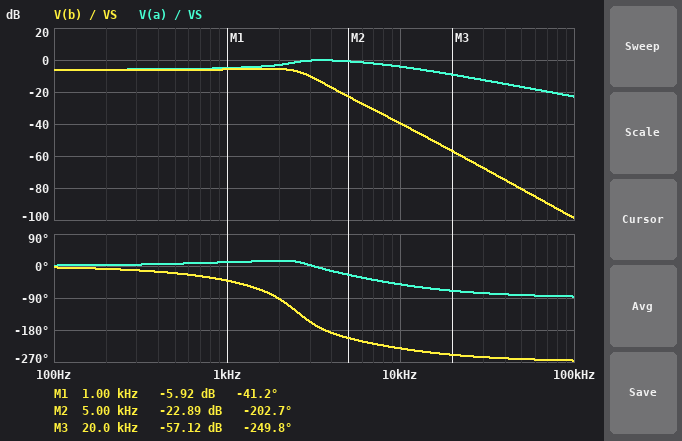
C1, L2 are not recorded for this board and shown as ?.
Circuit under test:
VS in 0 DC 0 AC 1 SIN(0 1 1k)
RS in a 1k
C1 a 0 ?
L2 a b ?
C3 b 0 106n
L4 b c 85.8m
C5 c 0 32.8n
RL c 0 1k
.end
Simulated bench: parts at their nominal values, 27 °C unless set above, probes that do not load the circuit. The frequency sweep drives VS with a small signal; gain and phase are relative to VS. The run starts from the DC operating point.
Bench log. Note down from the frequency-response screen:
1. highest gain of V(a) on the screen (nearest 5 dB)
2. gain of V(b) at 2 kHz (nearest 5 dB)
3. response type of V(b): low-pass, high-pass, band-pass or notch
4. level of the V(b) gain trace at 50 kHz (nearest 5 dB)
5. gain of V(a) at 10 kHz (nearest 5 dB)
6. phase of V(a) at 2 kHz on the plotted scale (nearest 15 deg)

0 dB
-5 dB
low-pass
-80 dB
-5 dB
15 deg
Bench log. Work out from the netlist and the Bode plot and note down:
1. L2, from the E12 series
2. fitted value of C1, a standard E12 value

150 mH
22 nF
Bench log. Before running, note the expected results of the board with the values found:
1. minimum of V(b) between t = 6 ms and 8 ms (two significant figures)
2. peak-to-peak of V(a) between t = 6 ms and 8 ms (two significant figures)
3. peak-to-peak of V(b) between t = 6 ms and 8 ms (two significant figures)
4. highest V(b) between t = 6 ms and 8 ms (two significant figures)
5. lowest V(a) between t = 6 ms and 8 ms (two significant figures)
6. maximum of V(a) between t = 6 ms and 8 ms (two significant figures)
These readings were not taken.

-510 mV
1.1 V
1.0 V
510 mV
-560 mV
560 mV
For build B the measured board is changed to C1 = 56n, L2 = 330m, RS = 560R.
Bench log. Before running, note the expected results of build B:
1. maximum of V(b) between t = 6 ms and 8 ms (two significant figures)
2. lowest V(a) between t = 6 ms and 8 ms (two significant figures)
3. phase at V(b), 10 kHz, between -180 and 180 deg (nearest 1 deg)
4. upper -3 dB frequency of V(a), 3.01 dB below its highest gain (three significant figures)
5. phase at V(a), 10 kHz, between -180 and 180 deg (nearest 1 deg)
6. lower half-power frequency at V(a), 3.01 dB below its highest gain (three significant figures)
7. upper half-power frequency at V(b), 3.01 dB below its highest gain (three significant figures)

450 mV
-880 mV
117 deg
5.88 kHz
-63 deg
223 Hz
995 Hz
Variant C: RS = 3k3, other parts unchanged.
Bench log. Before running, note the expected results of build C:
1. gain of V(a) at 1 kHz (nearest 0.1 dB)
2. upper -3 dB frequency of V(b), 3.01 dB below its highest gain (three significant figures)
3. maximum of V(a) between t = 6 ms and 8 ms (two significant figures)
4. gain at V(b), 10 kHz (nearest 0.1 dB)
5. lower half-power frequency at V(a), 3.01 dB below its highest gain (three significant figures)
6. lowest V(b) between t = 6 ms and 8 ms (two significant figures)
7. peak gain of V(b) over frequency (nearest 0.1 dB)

-11.3 dB
3.33 kHz
270 mV
-48.3 dB
2.61 kHz
-250 mV
-10.1 dB
